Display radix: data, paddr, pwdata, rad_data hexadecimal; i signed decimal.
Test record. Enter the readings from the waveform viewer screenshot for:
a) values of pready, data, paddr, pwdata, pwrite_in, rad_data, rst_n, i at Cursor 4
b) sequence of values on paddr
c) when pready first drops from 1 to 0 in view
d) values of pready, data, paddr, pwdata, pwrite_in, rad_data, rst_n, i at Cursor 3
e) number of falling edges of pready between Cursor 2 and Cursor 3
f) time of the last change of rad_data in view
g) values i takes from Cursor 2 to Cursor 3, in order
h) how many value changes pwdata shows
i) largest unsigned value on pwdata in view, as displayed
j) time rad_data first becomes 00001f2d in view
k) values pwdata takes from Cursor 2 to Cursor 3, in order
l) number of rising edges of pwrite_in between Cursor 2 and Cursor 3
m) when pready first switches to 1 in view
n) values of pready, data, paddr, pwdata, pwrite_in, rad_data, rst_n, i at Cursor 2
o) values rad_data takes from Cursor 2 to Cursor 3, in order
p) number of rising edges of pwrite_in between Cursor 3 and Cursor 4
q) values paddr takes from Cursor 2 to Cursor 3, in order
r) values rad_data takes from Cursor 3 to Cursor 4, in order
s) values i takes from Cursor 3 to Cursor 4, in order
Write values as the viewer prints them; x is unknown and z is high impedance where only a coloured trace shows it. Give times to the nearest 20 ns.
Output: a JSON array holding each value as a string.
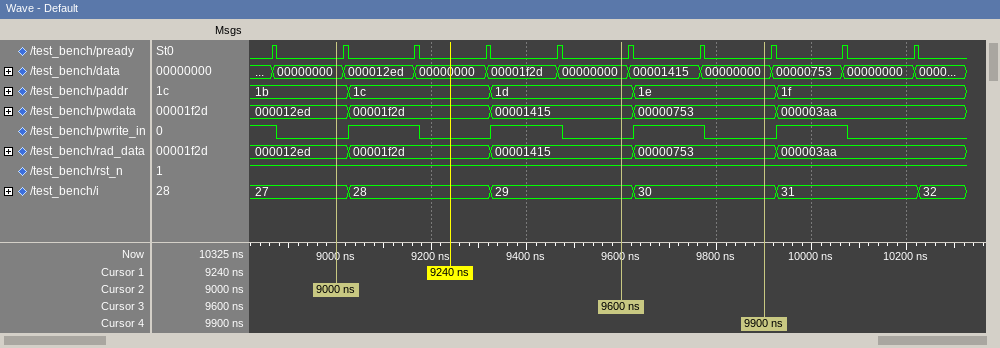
["pready=0, data=00000000, paddr=1e, pwdata=00000753, pwrite_in=0, rad_data=00000753, rst_n=1, i=30", "1b, 1c, 1d, 1e, 1f", "8880 ns", "pready=0, data=00000000, paddr=1d, pwdata=00001415, pwrite_in=0, rad_data=00001415, rst_n=1, i=29", "4", "9920 ns", "27, 28, 29", "4", "00001f2d", "9020 ns", "000012ed, 00001f2d, 00001415", "2", "8860 ns", "pready=0, data=00000000, paddr=1b, pwdata=000012ed, pwrite_in=0, rad_data=000012ed, rst_n=1, i=27", "000012ed, 00001f2d, 00001415", "1", "1b, 1c, 1d", "00001415, 00000753", "29, 30"]
